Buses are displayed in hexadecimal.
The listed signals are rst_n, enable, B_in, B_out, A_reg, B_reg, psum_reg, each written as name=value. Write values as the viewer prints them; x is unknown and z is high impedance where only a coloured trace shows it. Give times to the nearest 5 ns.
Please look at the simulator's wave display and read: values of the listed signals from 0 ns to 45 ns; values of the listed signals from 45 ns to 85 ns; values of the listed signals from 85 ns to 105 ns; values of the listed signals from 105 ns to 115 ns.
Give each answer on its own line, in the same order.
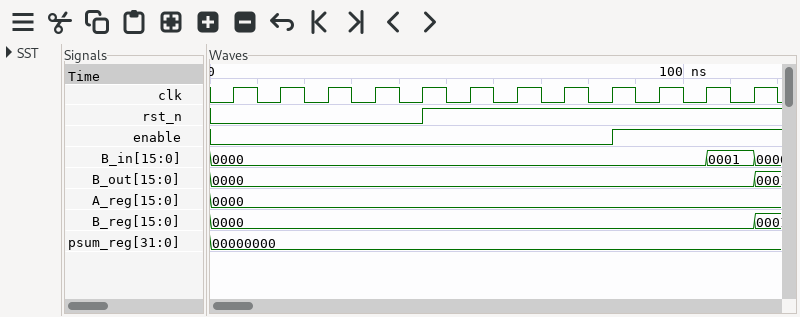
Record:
rst_n=0, enable=0, B_in=0000, B_out=0000, A_reg=0000, B_reg=0000, psum_reg=00000000
rst_n=1, enable=0, B_in=0000, B_out=0000, A_reg=0000, B_reg=0000, psum_reg=00000000
rst_n=1, enable=1, B_in=0000, B_out=0000, A_reg=0000, B_reg=0000, psum_reg=00000000
rst_n=1, enable=1, B_in=0001, B_out=0000, A_reg=0000, B_reg=0000, psum_reg=00000000
